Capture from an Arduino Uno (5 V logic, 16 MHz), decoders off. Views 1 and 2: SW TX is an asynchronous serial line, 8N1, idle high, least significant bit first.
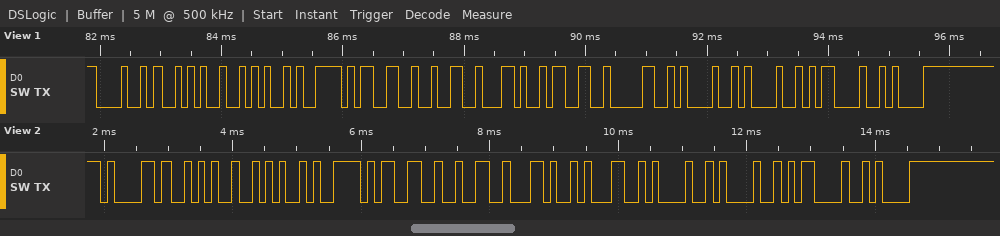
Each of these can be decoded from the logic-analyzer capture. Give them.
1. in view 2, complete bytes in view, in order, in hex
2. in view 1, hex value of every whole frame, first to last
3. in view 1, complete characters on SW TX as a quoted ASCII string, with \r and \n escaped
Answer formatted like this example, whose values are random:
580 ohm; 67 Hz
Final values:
61 2A 2A 79 33 32 2C 31 21 21 0D 0A; 0x48 0x2A 0x2A 0x79 0x33 0x32 0x2C 0x33 0x30 0x21 0x21 0x0D 0x0A; "H**y32,30!!\r\n"
